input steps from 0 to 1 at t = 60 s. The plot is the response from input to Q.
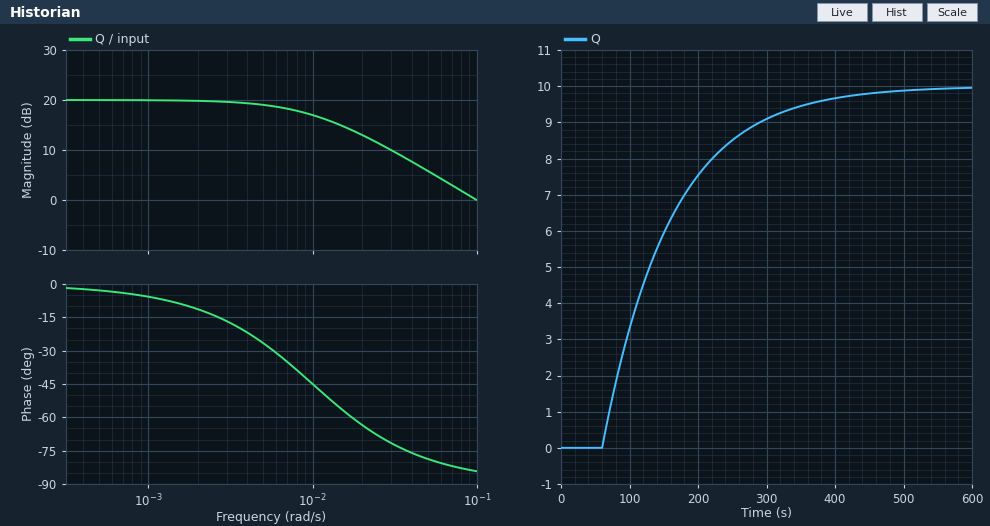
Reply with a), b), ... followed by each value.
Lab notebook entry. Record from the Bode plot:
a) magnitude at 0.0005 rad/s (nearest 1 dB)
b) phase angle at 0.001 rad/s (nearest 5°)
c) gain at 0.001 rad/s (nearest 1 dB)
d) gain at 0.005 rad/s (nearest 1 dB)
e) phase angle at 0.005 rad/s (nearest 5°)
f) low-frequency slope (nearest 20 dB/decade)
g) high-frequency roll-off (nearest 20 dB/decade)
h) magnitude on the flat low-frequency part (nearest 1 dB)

a) 20 dB
b) -5°
c) 20 dB
d) 19 dB
e) -25°
f) 0 dB/decade
g) -20 dB/decade
h) 20 dB
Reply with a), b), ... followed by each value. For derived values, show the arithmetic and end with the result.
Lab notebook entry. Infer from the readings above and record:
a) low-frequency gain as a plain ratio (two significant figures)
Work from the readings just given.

a) 10^(20 / 20) = 10
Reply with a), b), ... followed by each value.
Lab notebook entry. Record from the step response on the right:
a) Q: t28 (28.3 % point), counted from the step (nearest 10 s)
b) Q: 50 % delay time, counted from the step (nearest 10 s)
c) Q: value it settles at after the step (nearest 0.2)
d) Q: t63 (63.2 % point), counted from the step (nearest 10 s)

a) 30 s
b) 70 s
c) 10.0
d) 100 s
